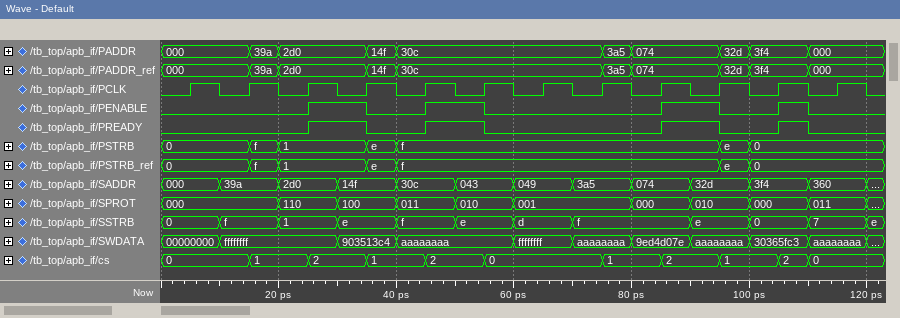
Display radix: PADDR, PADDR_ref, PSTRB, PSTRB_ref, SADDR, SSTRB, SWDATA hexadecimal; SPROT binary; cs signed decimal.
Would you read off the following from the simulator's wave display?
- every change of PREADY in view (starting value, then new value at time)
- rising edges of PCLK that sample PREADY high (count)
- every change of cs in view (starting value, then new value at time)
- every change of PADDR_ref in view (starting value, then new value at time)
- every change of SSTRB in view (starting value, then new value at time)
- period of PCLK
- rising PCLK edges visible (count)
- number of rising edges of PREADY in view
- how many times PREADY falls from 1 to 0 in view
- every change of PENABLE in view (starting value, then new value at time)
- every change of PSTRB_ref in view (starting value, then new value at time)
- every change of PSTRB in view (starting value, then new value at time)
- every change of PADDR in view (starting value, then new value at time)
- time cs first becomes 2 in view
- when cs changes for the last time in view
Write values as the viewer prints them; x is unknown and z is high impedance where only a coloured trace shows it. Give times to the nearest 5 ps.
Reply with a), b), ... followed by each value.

a) 0, 1 at 25 ps, 0 at 35 ps, 1 at 45 ps, 0 at 55 ps, 1 at 85 ps, 0 at 95 ps, 1 at 105 ps, 0 at 110 ps
b) 3
c) 0, 1 at 15 ps, 2 at 25 ps, 1 at 35 ps, 2 at 45 ps, 0 at 55 ps, 1 at 75 ps, 2 at 85 ps, 1 at 95 ps, 2 at 105 ps, 0 at 110 ps
d) 000, 39a at 15 ps, 2d0 at 20 ps, 14f at 35 ps, 30c at 40 ps, 3a5 at 75 ps, 074 at 80 ps, 32d at 95 ps, 3f4 at 100 ps, 000 at 110 ps
e) 0, f at 10 ps, 1 at 20 ps, e at 30 ps, f at 40 ps, e at 50 ps, d at 60 ps, f at 70 ps, e at 90 ps, 0 at 100 ps, 7 at 110 ps, e at 120 ps
f) 10 ps
g) 12
h) 4
i) 4
j) 0, 1 at 25 ps, 0 at 35 ps, 1 at 45 ps, 0 at 55 ps, 1 at 85 ps, 0 at 95 ps, 1 at 105 ps, 0 at 110 ps
k) 0, f at 15 ps, 1 at 20 ps, e at 35 ps, f at 40 ps, e at 95 ps, 0 at 100 ps
l) 0, f at 15 ps, 1 at 20 ps, e at 35 ps, f at 40 ps, e at 95 ps, 0 at 100 ps
m) 000, 39a at 15 ps, 2d0 at 20 ps, 14f at 35 ps, 30c at 40 ps, 3a5 at 75 ps, 074 at 80 ps, 32d at 95 ps, 3f4 at 100 ps, 000 at 110 ps
n) 25 ps
o) 110 ps
